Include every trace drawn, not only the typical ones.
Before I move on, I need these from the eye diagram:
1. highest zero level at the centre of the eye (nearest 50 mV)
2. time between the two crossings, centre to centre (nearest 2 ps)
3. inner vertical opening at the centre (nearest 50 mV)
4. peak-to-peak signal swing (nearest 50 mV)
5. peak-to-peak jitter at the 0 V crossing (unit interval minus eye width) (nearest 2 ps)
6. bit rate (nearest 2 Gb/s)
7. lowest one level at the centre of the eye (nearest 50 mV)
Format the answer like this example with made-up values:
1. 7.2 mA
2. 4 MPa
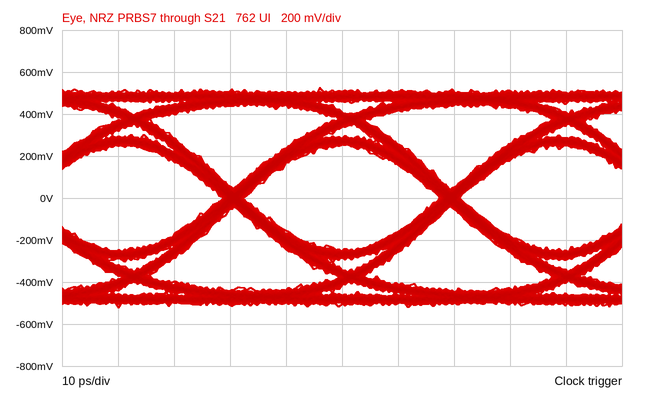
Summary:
1. -250 mV
2. 38 ps
3. 500 mV
4. 1.05 V
5. 4 ps
6. 26 Gb/s
7. 250 mV
